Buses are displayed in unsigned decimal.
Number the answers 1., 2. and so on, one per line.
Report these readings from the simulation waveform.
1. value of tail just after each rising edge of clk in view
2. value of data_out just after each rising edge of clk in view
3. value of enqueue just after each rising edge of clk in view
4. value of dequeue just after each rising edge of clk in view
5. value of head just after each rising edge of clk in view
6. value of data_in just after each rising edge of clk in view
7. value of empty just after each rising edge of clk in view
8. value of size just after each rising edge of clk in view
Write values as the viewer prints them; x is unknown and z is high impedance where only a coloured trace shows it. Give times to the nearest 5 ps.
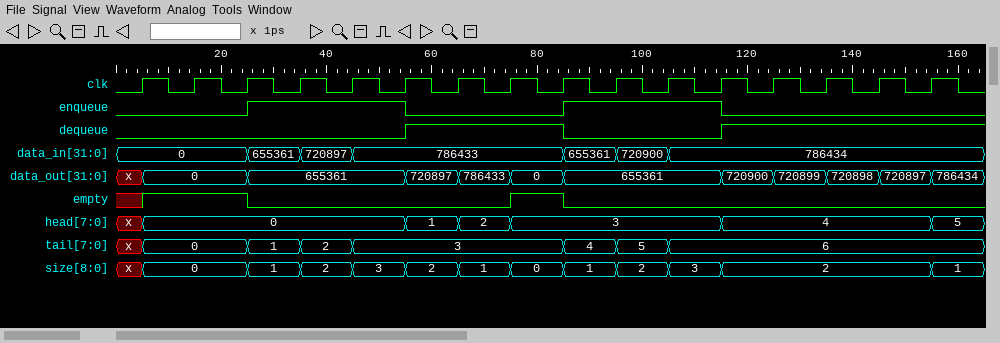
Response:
1. 0, 0, 1, 2, 3, 3, 3, 3, 4, 5, 6, 6, 6, 6, 6, 6
2. 0, 0, 655361, 655361, 655361, 720897, 786433, 0, 655361, 655361, 655361, 720900, 720899, 720898, 720897, 786434
3. 0 0 1 1 1 0 0 0 1 1 1 0 0 0 0 0
4. 0 0 0 0 0 1 1 1 0 0 0 1 1 1 1 1
5. 0, 0, 0, 0, 0, 1, 2, 3, 3, 3, 3, 4, 4, 4, 4, 5
6. 0, 0, 655361, 720897, 786433, 786433, 786433, 786433, 655361, 720900, 786434, 786434, 786434, 786434, 786434, 786434
7. 1 1 0 0 0 0 0 1 0 0 0 0 0 0 0 0
8. 0, 0, 1, 2, 3, 2, 1, 0, 1, 2, 3, 2, 2, 2, 2, 1
